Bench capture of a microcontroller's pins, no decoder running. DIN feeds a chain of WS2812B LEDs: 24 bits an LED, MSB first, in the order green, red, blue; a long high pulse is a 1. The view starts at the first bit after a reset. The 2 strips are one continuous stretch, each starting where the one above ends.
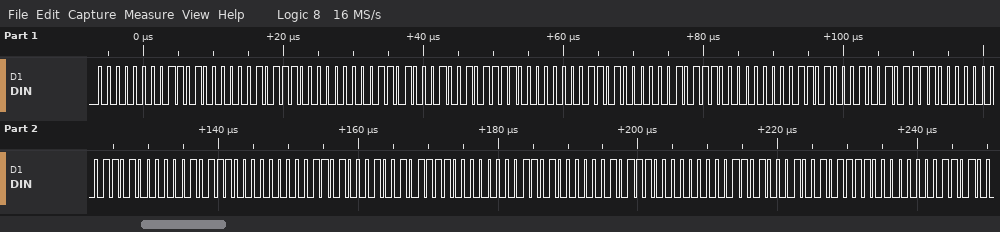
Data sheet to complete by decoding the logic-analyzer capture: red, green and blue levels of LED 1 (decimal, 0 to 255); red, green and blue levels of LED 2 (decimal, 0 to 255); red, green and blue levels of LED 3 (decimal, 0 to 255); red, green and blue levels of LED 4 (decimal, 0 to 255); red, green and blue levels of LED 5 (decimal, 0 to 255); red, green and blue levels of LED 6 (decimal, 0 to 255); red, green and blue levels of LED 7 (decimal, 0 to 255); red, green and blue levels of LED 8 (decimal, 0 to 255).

208, 0, 46
209, 0, 47
208, 0, 46
209, 0, 47
208, 0, 46
209, 0, 47
208, 0, 46
209, 0, 47
